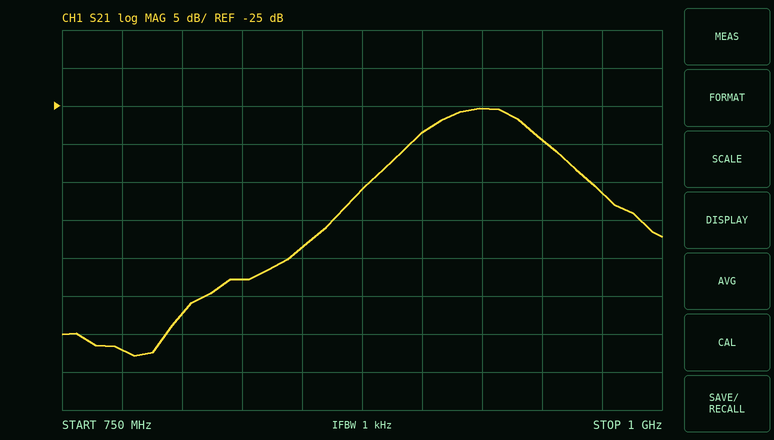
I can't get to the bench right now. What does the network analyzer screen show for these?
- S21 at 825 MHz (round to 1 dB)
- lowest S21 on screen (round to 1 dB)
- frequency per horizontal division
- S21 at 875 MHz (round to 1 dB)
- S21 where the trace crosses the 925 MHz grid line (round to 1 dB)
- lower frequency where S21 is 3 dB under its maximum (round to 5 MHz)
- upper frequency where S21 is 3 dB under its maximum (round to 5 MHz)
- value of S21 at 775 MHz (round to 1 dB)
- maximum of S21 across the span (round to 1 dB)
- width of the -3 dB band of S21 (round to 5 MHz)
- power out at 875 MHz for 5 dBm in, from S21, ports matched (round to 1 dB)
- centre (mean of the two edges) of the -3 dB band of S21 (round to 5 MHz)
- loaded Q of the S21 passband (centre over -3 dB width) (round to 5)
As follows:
-48 dB
-58 dB
25 MHz
-36 dB
-25 dB
900 MHz
945 MHz
-57 dB
-25 dB
45 MHz
-31 dBm
925 MHz
20
